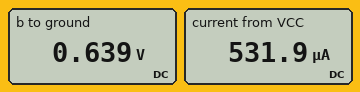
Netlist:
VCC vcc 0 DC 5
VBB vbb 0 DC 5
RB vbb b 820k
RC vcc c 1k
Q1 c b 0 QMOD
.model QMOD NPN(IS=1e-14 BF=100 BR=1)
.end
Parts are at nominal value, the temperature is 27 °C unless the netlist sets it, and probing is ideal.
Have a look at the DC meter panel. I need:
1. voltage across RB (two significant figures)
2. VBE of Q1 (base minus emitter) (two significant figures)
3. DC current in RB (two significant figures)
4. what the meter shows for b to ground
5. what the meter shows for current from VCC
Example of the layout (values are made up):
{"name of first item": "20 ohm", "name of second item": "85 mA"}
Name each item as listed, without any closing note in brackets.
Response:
{"voltage across RB": "4.4 V", "VBE of Q1 (base minus emitter)": "640 mV", "DC current in RB": "5.3 µA", "what the meter shows for b to ground": "0.639 V", "what the meter shows for current from VCC": "531.9 µA"}
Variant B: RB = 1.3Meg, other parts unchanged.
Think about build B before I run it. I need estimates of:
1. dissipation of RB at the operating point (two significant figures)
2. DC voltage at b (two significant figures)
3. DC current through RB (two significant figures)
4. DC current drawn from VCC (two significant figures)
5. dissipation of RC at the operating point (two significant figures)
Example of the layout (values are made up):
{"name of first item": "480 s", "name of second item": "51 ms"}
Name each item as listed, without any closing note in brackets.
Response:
{"dissipation of RB at the operating point": "15 µW", "DC voltage at b": "630 mV", "DC current through RB": "3.4 µA", "DC current drawn from VCC": "340 µA", "dissipation of RC at the operating point": "110 µW"}
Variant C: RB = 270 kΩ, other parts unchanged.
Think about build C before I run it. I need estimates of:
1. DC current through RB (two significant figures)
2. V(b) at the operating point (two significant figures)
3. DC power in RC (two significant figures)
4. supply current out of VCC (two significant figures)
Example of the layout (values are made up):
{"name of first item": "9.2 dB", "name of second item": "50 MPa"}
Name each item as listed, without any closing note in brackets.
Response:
{"DC current through RB": "16 µA", "V(b) at the operating point": "670 mV", "DC power in RC": "2.6 mW", "supply current out of VCC": "1.6 mA"}
